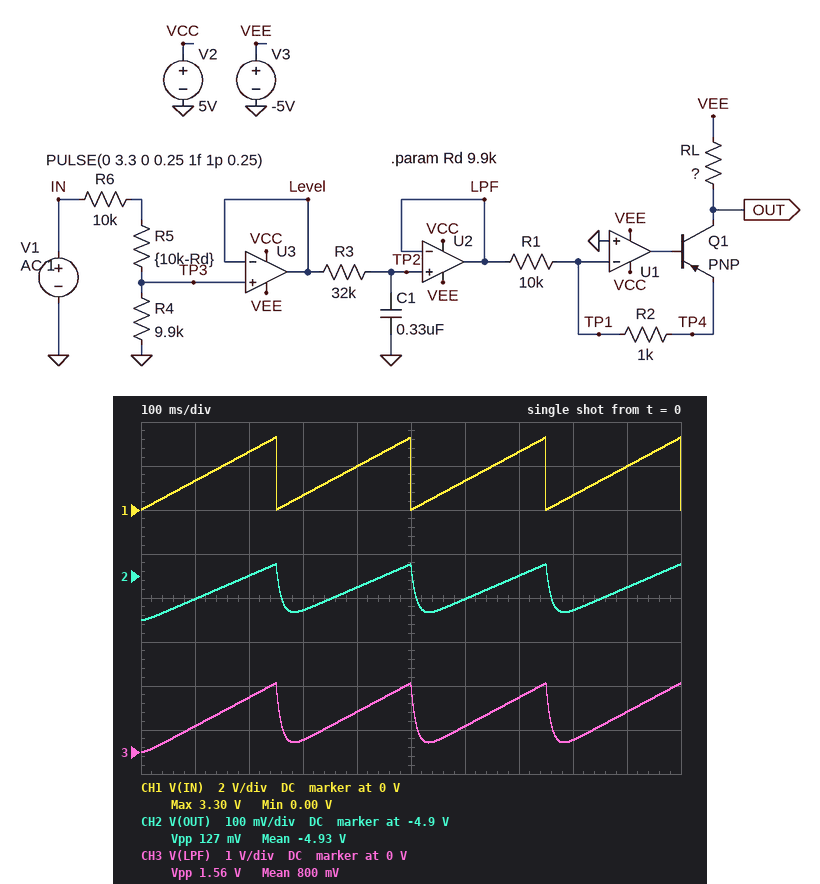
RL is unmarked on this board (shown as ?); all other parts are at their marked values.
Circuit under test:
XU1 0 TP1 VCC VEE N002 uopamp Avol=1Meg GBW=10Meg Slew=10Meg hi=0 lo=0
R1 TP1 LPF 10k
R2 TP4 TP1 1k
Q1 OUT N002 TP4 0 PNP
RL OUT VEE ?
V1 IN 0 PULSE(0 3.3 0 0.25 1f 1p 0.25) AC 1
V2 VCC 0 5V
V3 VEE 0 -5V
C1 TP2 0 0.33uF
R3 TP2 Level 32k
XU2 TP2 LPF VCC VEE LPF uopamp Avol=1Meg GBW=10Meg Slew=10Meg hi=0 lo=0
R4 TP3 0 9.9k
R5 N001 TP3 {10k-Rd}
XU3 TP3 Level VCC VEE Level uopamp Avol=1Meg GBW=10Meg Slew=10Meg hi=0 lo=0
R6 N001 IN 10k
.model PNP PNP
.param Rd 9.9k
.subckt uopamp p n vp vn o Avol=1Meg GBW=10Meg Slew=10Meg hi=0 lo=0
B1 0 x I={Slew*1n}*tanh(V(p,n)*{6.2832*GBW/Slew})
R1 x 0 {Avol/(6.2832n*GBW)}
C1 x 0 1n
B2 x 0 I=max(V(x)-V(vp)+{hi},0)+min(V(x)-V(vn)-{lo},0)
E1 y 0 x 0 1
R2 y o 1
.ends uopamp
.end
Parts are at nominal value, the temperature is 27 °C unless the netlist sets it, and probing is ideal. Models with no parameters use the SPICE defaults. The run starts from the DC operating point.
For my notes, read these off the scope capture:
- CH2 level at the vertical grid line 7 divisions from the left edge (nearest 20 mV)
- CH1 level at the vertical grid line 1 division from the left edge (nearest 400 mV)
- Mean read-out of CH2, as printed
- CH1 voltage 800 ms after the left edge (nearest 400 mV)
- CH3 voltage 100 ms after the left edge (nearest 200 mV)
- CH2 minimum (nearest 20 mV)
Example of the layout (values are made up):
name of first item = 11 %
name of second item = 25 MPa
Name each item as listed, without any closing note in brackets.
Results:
CH2 level at the vertical grid line 7 divisions from the left edge = -4.90 V
CH1 level at the vertical grid line 1 division from the left edge = 1.2 V
Mean read-out of CH2, as printed = -4.93 V
CH1 voltage 800 ms after the left edge = 800 mV
CH3 voltage 100 ms after the left edge = 600 mV
CH2 minimum = -5.00 V
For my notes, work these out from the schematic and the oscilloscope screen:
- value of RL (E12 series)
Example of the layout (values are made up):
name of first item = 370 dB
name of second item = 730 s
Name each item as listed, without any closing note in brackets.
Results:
value of RL = 820 Ω
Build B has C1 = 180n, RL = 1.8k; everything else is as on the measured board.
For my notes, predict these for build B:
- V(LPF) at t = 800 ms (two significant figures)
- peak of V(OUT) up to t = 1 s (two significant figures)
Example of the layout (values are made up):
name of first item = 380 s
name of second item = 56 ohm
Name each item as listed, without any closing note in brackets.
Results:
V(LPF) at t = 800 ms = 290 mV
peak of V(OUT) up to t = 1 s = -4.7 V
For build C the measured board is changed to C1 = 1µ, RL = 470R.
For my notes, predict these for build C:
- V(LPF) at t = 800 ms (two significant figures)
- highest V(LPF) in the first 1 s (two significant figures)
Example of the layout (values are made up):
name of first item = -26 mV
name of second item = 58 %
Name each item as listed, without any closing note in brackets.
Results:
V(LPF) at t = 800 ms = 460 mV
highest V(LPF) in the first 1 s = 1.4 V
